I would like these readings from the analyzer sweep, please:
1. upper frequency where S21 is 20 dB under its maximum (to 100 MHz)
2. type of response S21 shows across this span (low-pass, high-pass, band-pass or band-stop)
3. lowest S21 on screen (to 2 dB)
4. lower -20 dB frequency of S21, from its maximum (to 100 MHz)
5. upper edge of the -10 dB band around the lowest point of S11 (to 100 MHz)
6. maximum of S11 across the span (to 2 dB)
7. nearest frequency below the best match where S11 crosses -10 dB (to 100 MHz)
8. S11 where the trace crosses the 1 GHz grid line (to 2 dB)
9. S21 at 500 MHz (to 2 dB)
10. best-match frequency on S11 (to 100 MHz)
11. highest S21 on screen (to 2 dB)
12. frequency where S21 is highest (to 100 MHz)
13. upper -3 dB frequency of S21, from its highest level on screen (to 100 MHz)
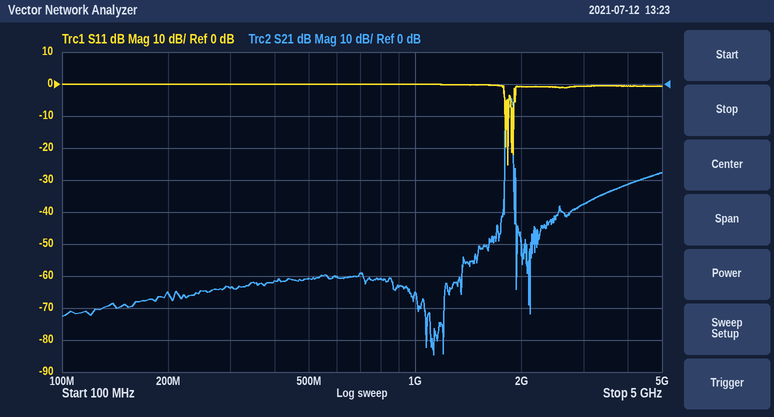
1.9 GHz
band-pass
-84 dB
1.8 GHz
1.8 GHz
0 dB
1.8 GHz
0 dB
-60 dB
1.8 GHz
-4 dB
1.9 GHz
1.9 GHz
